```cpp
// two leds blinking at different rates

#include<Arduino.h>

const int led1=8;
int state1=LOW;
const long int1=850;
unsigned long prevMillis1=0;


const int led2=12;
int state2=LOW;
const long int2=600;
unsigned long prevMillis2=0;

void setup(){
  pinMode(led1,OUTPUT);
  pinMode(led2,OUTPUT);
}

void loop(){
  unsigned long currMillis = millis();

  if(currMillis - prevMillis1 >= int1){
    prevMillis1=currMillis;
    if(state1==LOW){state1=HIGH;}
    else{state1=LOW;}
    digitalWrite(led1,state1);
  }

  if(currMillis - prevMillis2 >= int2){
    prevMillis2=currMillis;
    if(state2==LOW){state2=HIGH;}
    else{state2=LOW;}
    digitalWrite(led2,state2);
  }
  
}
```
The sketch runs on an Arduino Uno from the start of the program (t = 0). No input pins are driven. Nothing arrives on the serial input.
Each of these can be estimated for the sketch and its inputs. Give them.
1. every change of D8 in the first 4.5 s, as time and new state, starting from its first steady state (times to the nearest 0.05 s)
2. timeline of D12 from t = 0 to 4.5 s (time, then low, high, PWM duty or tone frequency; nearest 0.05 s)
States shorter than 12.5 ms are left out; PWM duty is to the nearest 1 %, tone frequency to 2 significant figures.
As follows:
0 s low; 0.85 s high; 1.7 s low; 2.55 s high; 3.4 s low; 4.25 s high
0 s low; 0.6 s high; 1.2 s low; 1.8 s high; 2.4 s low; 3 s high; 3.6 s low; 4.2 s high
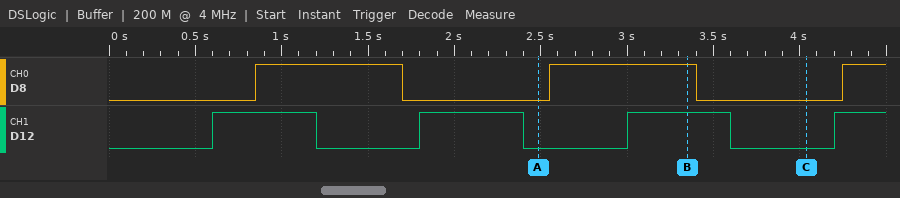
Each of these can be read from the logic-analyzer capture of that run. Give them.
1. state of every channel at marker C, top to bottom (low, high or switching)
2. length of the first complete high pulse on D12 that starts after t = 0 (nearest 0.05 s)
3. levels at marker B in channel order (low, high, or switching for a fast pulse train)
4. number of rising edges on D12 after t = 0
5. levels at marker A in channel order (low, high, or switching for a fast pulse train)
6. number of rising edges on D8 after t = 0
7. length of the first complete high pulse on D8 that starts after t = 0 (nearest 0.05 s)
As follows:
D8 low, D12 low
0.60 s
D8 high, D12 high
4
D8 low, D12 low
3
0.85 s
